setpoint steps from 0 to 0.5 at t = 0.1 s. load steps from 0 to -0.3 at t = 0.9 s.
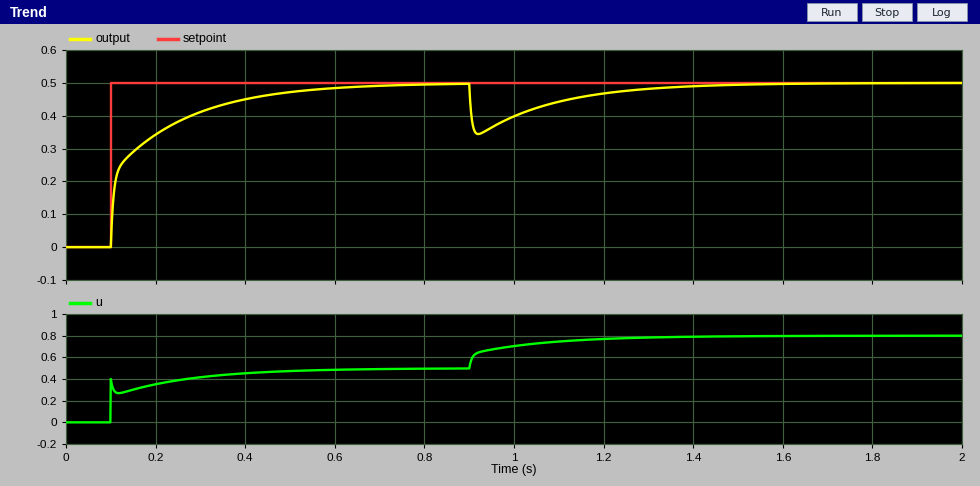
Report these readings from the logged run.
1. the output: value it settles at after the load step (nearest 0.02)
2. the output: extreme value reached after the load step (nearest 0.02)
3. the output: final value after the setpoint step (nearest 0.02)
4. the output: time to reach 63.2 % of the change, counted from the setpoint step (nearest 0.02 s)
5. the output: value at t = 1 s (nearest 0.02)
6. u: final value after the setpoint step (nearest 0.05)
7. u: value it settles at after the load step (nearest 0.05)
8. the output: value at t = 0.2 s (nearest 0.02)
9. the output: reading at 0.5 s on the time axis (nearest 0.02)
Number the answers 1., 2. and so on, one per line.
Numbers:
1. 0.50
2. 0.34
3. 0.50
4. 0.08 s
5. 0.40
6. 0.50
7. 0.80
8. 0.34
9. 0.48
